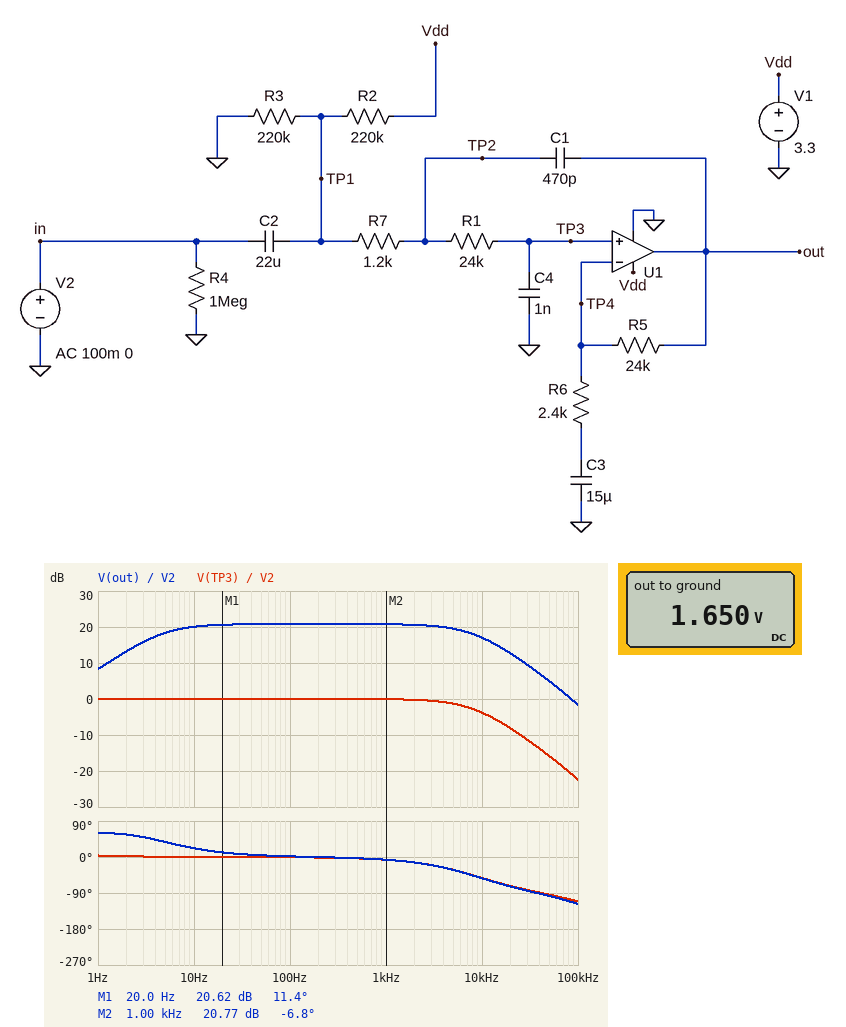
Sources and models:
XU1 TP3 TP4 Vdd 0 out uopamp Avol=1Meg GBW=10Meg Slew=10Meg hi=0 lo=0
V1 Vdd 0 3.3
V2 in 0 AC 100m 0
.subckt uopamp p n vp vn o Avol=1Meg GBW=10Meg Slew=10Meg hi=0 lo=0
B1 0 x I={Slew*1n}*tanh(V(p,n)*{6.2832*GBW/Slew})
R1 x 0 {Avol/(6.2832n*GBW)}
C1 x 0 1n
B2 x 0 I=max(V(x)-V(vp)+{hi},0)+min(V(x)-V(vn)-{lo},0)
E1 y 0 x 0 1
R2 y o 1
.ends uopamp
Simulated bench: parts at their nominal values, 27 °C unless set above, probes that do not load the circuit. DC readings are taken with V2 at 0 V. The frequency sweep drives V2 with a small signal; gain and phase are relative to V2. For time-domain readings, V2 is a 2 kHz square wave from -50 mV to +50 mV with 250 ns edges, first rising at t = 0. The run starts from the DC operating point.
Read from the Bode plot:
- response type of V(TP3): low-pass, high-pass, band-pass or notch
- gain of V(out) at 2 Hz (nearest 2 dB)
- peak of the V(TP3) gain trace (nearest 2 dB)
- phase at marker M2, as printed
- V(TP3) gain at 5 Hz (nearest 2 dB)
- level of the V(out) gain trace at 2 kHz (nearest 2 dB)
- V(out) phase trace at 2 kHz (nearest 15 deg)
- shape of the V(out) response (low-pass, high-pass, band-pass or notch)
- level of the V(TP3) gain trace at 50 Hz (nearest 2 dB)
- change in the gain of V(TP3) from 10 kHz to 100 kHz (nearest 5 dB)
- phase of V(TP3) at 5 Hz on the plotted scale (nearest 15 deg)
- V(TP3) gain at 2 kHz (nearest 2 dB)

low-pass
14 dB
0 dB
-6.8 deg
0 dB
20 dB
-15 deg
band-pass
0 dB
-20 dB
0 deg
0 dB
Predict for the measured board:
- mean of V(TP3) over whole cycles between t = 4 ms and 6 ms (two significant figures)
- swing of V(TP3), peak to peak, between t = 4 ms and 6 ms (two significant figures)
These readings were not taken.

1.7 V
100 mV
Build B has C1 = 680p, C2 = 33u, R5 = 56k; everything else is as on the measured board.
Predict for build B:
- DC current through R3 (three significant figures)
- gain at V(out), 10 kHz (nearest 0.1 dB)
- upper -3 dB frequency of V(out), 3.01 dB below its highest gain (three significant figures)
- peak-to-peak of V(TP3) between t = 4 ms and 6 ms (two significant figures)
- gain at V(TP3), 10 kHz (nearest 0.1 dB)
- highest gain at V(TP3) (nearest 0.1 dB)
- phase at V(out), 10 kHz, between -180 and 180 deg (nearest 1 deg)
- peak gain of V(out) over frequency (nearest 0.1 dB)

7.50 µA
28.0 dB
33.6 kHz
110 mV
0.2 dB
0.4 dB
-25 deg
28.1 dB
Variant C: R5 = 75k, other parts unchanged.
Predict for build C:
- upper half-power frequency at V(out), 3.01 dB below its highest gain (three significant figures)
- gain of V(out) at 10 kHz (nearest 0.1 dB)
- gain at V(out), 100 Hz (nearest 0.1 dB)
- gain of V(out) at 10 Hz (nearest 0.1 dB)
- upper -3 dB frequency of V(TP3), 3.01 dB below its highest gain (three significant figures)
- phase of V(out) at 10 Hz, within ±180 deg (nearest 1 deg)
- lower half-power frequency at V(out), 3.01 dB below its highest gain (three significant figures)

28.5 kHz
29.9 dB
30.2 dB
29.4 dB
28.6 kHz
23 deg
4.42 Hz
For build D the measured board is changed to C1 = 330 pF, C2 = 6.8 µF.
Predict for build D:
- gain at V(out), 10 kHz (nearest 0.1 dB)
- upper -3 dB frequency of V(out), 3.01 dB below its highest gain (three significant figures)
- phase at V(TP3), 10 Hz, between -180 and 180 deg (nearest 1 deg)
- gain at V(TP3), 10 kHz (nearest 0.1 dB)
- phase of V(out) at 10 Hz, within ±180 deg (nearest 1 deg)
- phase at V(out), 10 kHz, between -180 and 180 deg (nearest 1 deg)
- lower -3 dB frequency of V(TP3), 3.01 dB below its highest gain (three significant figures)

16.5 dB
7.67 kHz
1 deg
-4.3 dB
23 deg
-55 deg
213 mHz
